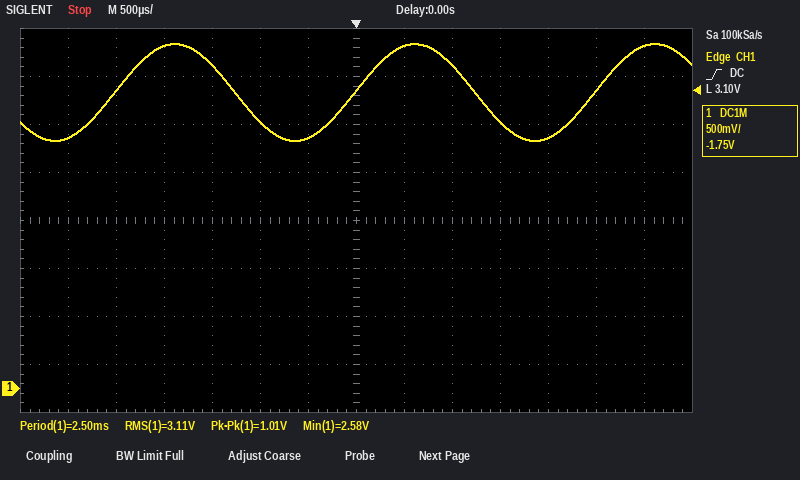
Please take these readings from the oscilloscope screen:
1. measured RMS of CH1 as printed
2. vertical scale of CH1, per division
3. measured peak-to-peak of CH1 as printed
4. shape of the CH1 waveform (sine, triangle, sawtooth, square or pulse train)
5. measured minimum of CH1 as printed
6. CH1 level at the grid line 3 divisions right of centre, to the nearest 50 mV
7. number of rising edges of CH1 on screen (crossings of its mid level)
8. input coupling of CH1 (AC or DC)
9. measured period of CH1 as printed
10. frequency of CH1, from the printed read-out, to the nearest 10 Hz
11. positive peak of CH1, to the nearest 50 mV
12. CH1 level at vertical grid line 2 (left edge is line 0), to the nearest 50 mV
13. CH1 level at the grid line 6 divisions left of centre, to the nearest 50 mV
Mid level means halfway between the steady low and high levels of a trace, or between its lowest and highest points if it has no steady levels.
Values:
3.11 V
500 mV
1.01 V
sine
2.58 V
2.80 V
3
DC
2.50 ms
400 Hz
3.60 V
3.10 V
2.60 V
